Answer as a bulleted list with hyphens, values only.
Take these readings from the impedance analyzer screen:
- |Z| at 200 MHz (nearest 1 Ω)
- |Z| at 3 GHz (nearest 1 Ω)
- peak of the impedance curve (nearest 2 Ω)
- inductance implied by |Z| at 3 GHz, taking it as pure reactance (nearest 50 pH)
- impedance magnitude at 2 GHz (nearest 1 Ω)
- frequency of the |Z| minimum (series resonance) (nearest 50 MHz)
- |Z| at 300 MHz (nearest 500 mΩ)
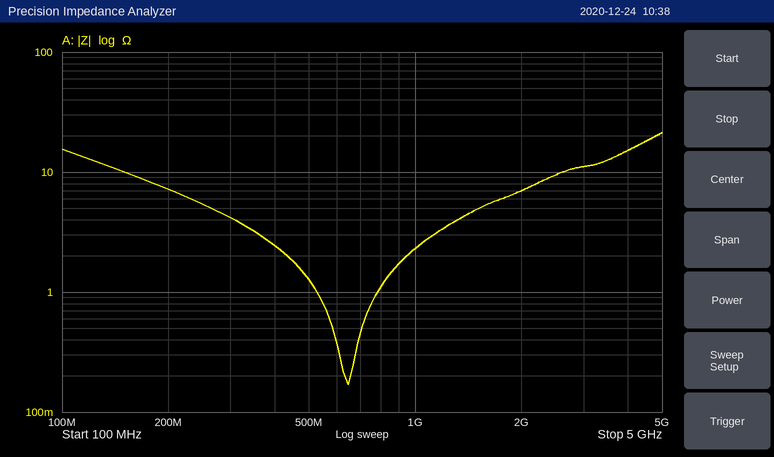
- 7 Ω
- 11 Ω
- 22 Ω
- 600 pH
- 7 Ω
- 650 MHz
- 4.0 Ω
